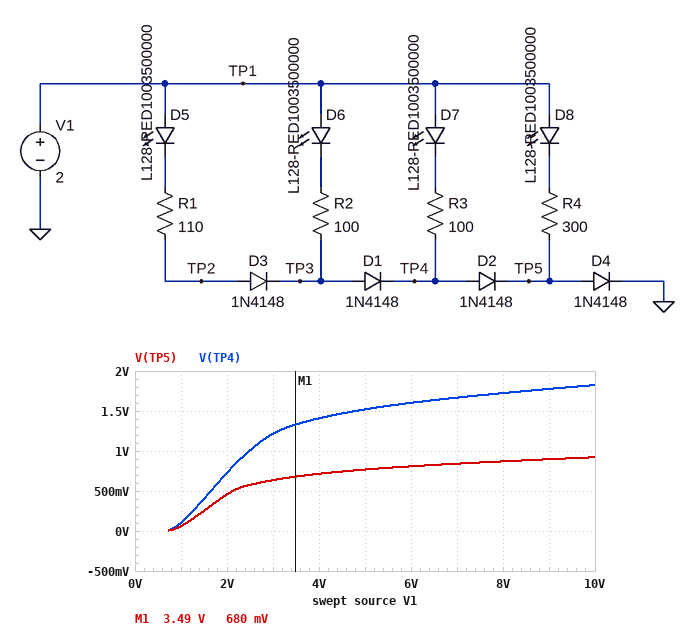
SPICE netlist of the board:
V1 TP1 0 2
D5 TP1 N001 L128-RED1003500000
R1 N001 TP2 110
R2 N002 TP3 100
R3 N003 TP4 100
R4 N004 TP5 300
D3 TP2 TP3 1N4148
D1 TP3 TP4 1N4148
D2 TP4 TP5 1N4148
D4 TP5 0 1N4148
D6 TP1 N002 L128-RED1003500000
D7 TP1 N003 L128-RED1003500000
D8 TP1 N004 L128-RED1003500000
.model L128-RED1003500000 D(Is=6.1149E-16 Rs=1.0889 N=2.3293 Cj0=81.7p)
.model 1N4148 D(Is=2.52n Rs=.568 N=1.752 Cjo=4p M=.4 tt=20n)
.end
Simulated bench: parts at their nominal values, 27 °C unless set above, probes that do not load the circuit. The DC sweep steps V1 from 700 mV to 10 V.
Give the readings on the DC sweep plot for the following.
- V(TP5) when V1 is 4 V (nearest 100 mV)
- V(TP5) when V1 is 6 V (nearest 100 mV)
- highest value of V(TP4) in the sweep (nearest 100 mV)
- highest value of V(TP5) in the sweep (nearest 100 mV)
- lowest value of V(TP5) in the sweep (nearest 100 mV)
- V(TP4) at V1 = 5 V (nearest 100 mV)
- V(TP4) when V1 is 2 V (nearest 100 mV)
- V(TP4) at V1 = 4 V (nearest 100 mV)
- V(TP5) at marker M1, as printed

700 mV
800 mV
1.8 V
900 mV
0 V
1.5 V
700 mV
1.4 V
680 mV
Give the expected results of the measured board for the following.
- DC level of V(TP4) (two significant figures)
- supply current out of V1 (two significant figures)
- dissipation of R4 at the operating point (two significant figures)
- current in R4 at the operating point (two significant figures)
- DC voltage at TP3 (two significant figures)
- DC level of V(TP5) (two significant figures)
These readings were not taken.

730 mV
61 µA
1.1 µW
60 µA
890 mV
460 mV
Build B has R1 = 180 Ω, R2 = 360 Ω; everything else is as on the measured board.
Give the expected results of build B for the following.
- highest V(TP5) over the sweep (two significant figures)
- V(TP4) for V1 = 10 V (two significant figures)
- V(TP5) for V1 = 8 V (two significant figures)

880 mV
1.7 V
840 mV
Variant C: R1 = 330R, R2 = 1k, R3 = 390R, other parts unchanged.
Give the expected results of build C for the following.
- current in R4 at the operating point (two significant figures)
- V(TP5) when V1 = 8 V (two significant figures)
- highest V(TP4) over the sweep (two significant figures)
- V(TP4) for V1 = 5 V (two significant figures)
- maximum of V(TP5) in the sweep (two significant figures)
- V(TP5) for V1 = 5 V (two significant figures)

60 µA
780 mV
1.6 V
1.4 V
810 mV
720 mV
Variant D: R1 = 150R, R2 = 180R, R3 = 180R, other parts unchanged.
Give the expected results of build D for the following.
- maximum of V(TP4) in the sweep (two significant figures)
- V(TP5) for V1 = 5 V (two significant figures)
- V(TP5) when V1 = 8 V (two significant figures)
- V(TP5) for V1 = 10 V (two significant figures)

1.7 V
750 mV
830 mV
870 mV
